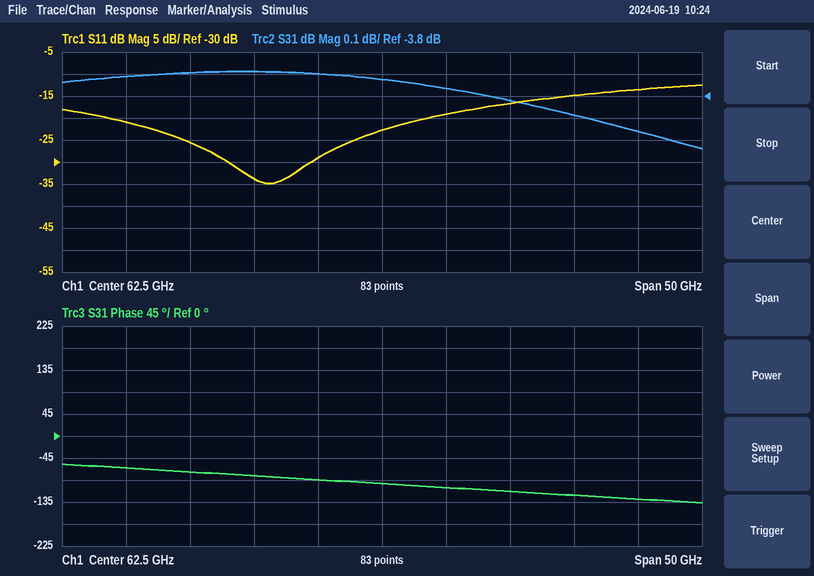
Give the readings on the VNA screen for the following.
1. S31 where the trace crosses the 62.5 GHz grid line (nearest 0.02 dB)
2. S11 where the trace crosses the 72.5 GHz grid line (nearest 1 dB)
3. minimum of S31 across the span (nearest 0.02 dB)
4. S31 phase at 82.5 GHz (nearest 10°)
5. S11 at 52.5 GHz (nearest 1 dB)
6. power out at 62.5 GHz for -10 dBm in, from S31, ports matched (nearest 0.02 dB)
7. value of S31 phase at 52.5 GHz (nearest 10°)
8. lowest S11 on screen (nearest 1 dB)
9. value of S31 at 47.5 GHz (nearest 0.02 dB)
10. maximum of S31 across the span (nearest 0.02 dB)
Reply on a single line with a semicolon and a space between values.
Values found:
-3.72 dB; -17 dB; -4.04 dB; -130°; -34 dB; -13.72 dBm; -80°; -35 dB; -3.70 dB; -3.68 dB
